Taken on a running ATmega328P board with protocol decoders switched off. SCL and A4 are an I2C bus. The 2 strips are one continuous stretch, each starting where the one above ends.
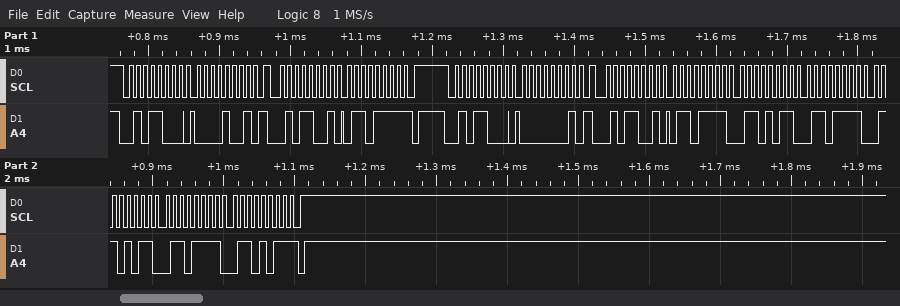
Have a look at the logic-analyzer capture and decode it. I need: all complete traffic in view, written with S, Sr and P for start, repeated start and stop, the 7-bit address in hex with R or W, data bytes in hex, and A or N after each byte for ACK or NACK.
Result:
S 2CW A 09 A Sr 2CR A 6F N P S 2CW A 01 A Sr 2CR A 6F A 6B A 6F A 6B A 6F A 6B N P
